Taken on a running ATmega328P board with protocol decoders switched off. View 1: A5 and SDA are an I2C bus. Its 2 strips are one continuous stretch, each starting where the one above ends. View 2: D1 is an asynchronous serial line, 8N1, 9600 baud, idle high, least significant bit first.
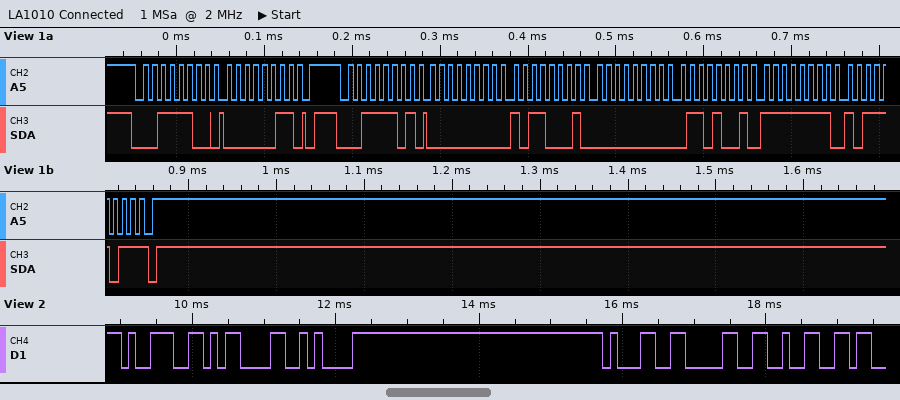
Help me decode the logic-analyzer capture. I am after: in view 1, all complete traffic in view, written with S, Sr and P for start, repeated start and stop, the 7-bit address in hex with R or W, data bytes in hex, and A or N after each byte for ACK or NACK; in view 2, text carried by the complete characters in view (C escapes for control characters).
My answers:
S 1EW A 03 A P S 1ER A 00 A B1 A 00 A 69 A FF A BB N P
"9\r\n102"
